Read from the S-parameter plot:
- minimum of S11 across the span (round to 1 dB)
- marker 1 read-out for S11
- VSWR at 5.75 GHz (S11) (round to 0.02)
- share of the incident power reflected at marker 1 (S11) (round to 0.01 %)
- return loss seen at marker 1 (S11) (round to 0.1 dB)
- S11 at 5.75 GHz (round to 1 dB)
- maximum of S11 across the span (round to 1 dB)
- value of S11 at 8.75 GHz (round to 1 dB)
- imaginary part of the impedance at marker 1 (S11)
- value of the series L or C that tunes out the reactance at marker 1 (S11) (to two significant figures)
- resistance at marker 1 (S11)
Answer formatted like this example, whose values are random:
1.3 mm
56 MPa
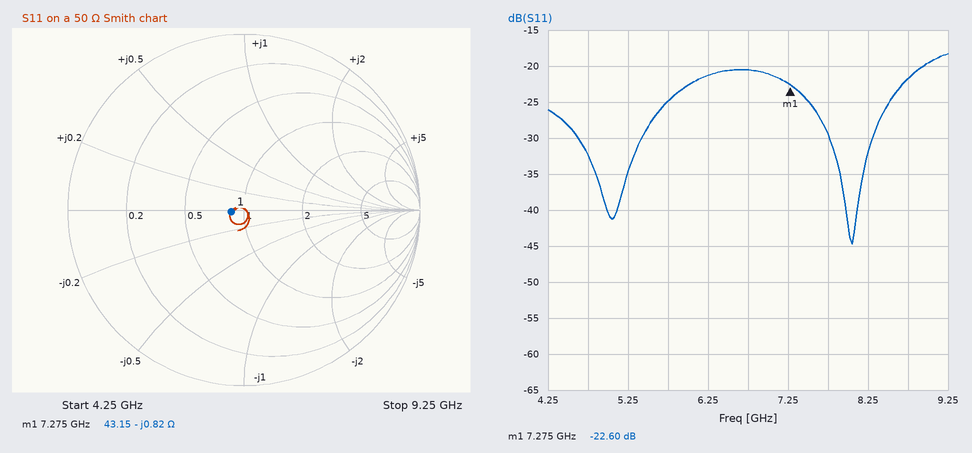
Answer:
-45 dB
-22.60 dB
1.12
0.55 %
22.6 dB
-25 dB
-18 dB
-22 dB
-0.82 Ω
18 pH
43.15 Ω
